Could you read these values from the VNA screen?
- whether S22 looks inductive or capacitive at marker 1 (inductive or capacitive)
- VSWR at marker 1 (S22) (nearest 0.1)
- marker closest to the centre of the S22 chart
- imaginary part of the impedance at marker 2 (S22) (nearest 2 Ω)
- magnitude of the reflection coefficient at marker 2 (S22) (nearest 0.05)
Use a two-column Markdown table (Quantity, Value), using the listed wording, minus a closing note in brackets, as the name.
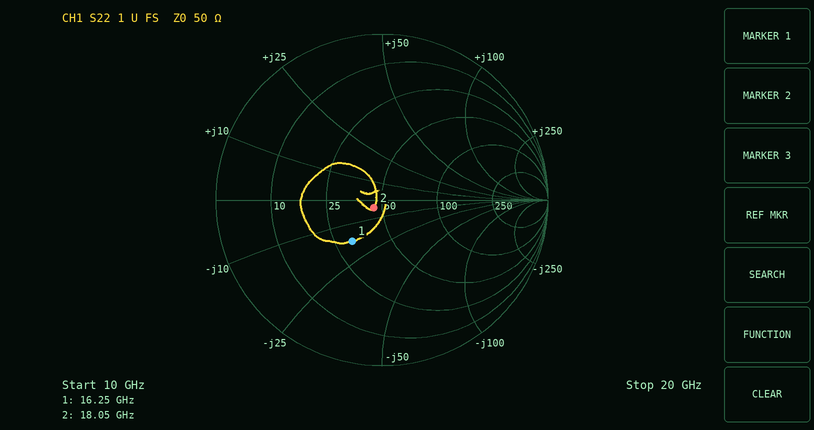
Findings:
| Quantity | Value |
|---|---|
| whether S22 looks inductive or capacitive at marker 1 | capacitive |
| VSWR at marker 1 (S22) | 1.9 |
| marker closest to the centre of the S22 chart | marker 2 |
| imaginary part of the impedance at marker 2 (S22) | -4 Ω |
| magnitude of the reflection coefficient at marker 2 (S22) | 0.05 |
